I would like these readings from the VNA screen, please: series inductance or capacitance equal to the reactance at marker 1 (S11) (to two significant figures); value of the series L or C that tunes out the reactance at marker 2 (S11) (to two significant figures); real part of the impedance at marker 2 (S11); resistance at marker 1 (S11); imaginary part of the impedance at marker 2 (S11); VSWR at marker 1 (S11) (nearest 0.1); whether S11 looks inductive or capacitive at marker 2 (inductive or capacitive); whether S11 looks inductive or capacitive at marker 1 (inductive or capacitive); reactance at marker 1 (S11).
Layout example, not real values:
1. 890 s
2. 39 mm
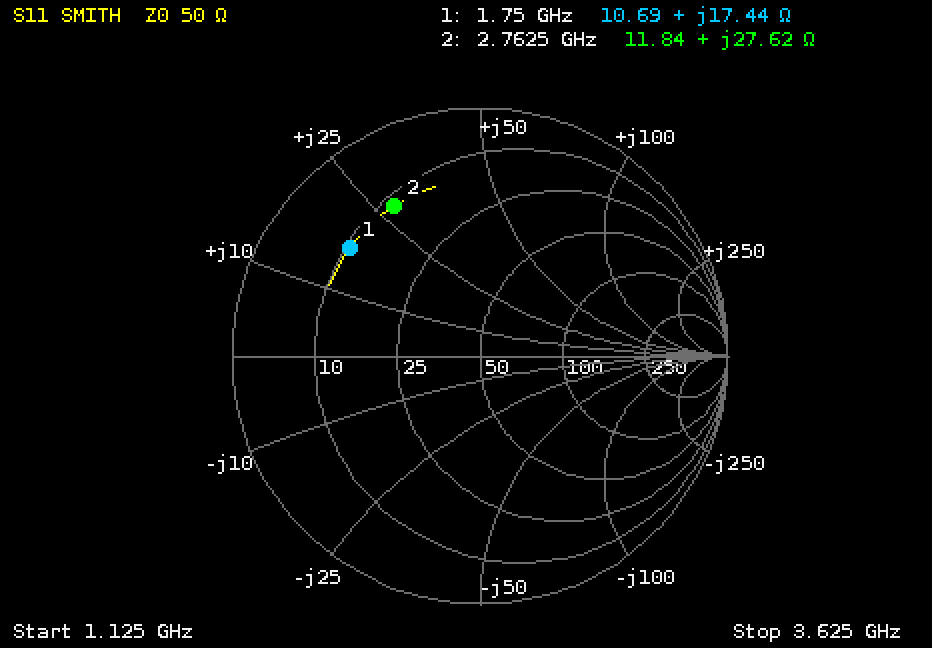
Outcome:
1. 1.6 nH
2. 2.1 pF
3. 11.84 Ω
4. 10.69 Ω
5. +27.62 Ω
6. 5.3
7. inductive
8. inductive
9. +17.44 Ω
